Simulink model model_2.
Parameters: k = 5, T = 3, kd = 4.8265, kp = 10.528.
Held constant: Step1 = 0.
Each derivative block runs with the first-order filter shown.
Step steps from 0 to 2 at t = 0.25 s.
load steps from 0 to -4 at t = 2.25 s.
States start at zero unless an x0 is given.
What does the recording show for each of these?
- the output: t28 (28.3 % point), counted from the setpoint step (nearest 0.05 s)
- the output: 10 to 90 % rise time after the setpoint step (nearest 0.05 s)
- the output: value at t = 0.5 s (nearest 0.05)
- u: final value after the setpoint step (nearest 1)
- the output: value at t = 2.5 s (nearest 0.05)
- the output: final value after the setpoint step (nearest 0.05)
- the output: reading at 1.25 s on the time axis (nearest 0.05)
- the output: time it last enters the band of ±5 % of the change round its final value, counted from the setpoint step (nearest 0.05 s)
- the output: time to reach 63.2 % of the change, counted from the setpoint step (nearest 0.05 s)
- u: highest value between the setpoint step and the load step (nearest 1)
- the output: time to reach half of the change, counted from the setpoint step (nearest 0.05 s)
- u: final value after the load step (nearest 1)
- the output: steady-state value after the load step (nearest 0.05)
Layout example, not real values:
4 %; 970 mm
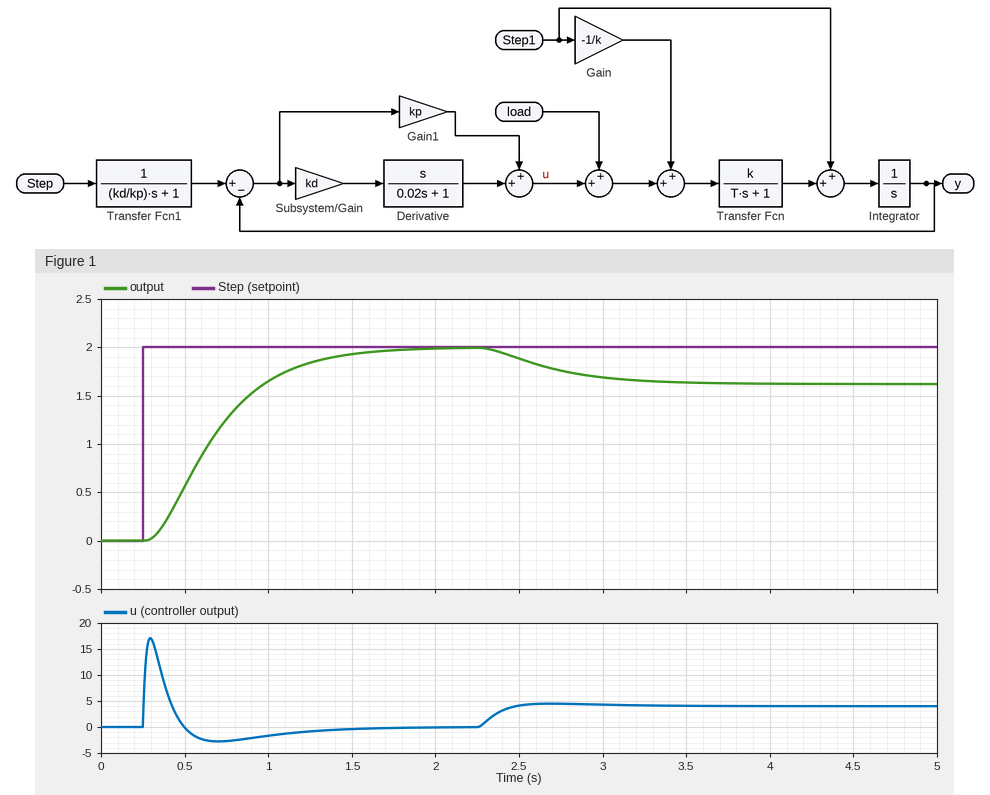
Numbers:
0.25 s; 0.80 s; 0.55; 0; 1.90; 2.00; 1.85; 1.15 s; 0.50 s; 17; 0.40 s; 4; 1.60
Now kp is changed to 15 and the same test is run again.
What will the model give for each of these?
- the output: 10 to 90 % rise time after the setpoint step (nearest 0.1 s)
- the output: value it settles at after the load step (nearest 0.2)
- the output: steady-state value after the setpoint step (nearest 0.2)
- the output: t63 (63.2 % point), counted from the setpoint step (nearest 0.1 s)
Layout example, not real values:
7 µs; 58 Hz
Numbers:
0.5 s; 1.8; 2.0; 0.4 s
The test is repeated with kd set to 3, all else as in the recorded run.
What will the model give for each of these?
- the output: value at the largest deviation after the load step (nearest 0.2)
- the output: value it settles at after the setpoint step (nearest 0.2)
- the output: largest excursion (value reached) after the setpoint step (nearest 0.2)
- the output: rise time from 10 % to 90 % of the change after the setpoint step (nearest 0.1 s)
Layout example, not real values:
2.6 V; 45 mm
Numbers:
1.6; 2.0; 2.2; 0.4 s
